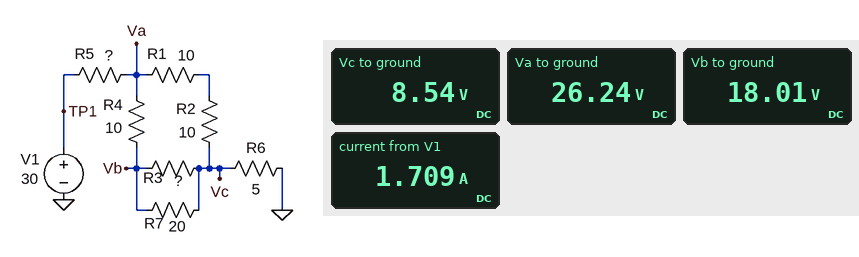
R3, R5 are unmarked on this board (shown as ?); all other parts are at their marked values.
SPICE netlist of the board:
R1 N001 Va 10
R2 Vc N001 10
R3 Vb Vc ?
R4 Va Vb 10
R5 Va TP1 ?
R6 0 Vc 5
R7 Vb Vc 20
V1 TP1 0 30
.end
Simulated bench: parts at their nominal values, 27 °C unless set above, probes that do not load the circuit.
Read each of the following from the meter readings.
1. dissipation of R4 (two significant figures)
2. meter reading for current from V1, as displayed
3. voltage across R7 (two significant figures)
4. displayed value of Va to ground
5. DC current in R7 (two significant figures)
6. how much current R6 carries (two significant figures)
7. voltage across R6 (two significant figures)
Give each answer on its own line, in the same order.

6.8 W
1.709 A
9.5 V
26.24 V
470 mA
1.7 A
8.5 V
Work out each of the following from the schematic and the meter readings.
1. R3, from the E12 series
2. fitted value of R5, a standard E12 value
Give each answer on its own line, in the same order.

27 Ω
2.2 Ω
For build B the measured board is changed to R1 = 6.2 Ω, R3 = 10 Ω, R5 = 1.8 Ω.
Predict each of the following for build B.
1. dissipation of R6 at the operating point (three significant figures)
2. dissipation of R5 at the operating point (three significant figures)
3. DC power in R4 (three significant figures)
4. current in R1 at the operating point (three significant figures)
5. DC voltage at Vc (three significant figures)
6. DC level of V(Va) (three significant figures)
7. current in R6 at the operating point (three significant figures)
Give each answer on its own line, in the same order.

20.0 W
7.19 W
9.70 W
1.01 A
9.99 V
26.4 V
2.00 A
